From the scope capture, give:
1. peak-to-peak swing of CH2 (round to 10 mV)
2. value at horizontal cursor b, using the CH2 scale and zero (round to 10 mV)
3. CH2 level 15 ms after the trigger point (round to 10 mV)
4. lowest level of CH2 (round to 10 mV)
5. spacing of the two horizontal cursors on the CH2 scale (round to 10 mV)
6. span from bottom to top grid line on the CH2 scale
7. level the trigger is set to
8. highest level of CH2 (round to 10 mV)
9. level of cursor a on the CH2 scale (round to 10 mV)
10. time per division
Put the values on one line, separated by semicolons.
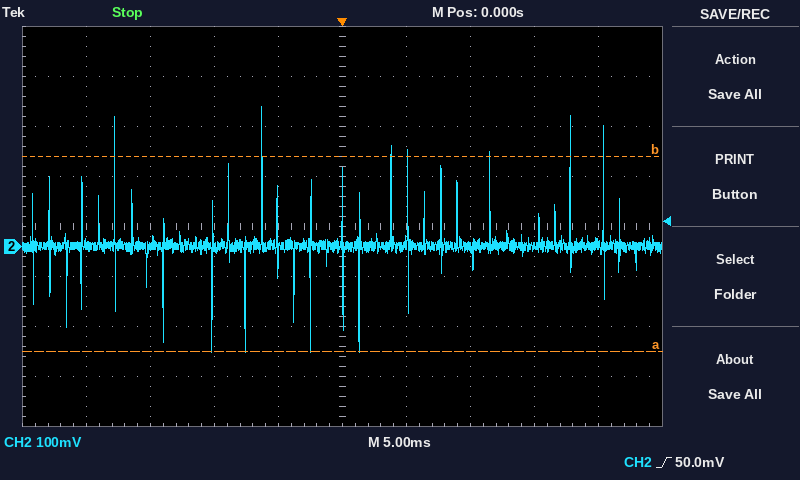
490 mV; 180 mV; 0 mV; -210 mV; 390 mV; 800 mV; 50.0 mV; 280 mV; -210 mV; 5 ms
